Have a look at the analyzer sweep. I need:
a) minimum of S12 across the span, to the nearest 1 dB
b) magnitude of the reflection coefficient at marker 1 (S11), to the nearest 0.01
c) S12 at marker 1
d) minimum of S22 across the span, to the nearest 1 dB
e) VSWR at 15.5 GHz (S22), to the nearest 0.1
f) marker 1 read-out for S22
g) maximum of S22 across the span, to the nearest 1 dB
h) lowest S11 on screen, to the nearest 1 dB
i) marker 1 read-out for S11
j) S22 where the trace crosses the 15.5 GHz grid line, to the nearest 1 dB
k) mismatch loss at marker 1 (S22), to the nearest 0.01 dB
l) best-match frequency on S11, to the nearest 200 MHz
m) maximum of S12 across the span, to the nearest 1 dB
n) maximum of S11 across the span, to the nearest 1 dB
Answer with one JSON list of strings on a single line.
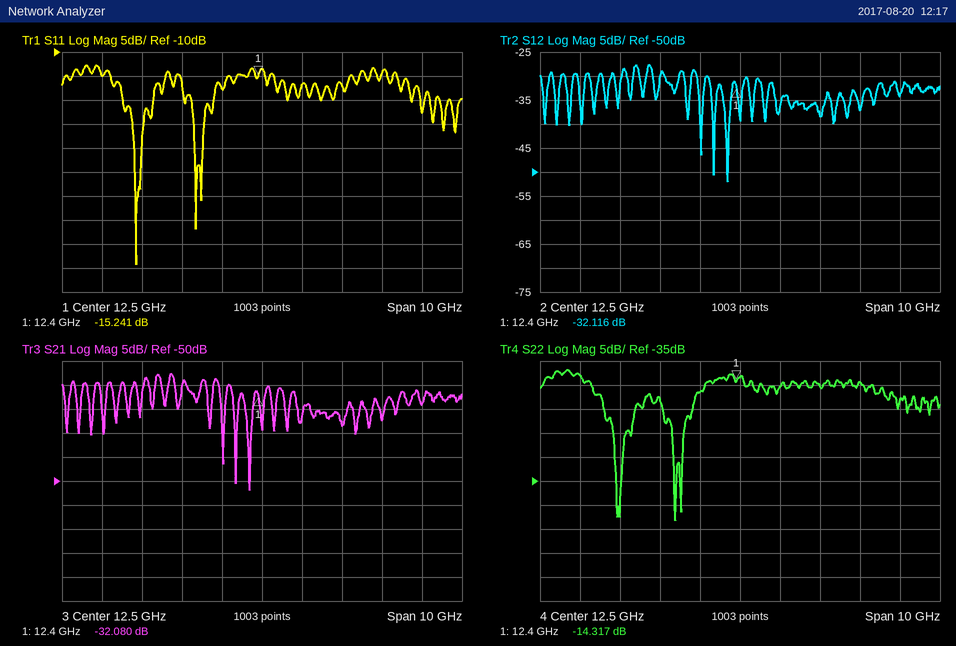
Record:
["-52 dB", "0.17", "-32.116 dB", "-43 dB", "1.5", "-14.317 dB", "-12 dB", "-54 dB", "-15.241 dB", "-14 dB", "0.16 dB", "9.4 GHz", "-28 dB", "-13 dB"]
